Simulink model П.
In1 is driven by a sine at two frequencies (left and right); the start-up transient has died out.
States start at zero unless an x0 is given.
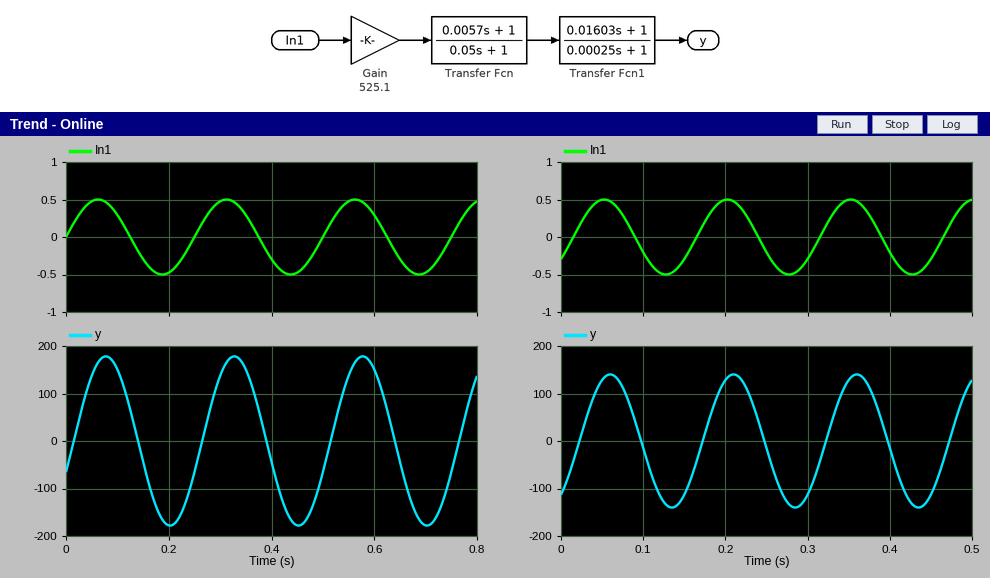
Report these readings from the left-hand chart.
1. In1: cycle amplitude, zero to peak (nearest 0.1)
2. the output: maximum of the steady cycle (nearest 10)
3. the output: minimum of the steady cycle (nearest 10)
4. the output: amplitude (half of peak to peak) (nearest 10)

0.5
180
-180
180
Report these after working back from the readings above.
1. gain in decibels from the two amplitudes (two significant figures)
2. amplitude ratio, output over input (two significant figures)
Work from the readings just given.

51 dB
360
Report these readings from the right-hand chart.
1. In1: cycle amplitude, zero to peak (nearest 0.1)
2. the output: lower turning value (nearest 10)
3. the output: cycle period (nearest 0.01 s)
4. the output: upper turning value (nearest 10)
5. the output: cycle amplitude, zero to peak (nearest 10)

0.5
-140
0.15 s
140
140
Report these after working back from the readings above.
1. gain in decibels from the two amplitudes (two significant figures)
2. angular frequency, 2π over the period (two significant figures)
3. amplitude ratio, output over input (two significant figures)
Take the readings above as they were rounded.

49 dB
42 rad/s
280
